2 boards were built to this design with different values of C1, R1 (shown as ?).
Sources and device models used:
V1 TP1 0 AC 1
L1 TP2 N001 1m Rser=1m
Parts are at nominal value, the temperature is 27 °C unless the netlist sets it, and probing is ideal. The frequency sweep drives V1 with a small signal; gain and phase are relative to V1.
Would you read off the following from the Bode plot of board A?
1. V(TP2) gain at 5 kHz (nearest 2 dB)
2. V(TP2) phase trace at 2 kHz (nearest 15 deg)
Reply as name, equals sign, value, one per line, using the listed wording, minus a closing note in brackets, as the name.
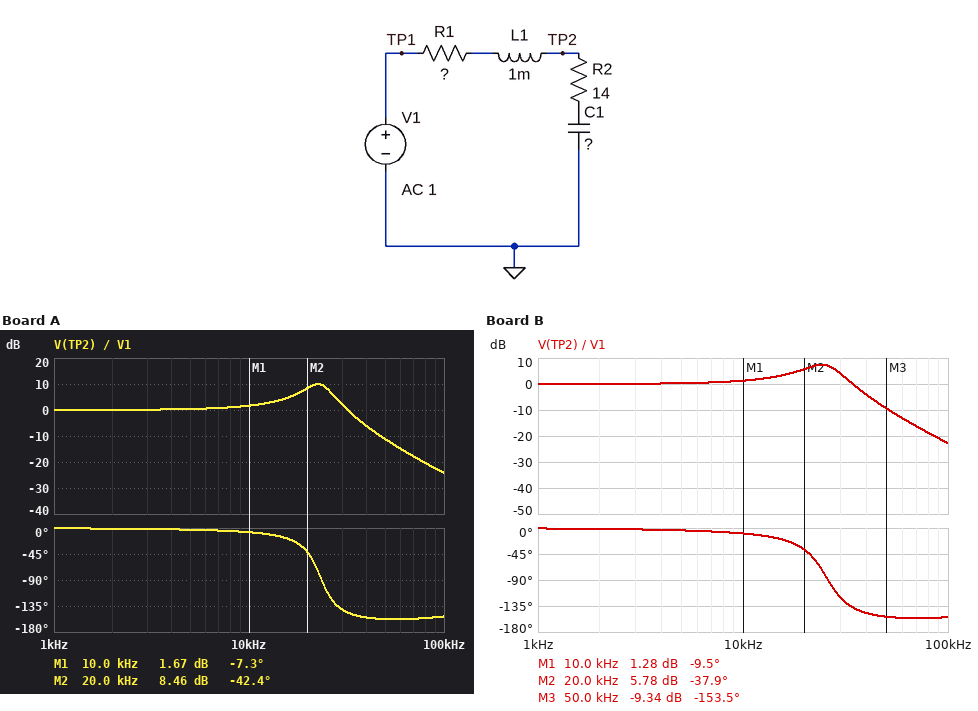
V(TP2) gain at 5 kHz = 0 dB
V(TP2) phase trace at 2 kHz = 0 deg
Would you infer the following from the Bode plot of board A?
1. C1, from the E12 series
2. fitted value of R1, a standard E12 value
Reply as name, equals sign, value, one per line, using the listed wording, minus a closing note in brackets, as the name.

C1, from the E12 series = 47 nF
fitted value of R1, a standard E12 value = 33 Ω
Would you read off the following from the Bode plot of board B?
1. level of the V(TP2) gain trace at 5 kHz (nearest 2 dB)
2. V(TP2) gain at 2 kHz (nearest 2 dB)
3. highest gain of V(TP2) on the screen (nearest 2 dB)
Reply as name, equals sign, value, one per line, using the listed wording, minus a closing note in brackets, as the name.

level of the V(TP2) gain trace at 5 kHz = 0 dB
V(TP2) gain at 2 kHz = 0 dB
highest gain of V(TP2) on the screen = 8 dB
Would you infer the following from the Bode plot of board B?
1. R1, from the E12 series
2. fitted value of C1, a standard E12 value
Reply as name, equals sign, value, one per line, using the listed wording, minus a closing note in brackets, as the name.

R1, from the E12 series = 56 Ω
fitted value of C1, a standard E12 value = 39 nF
